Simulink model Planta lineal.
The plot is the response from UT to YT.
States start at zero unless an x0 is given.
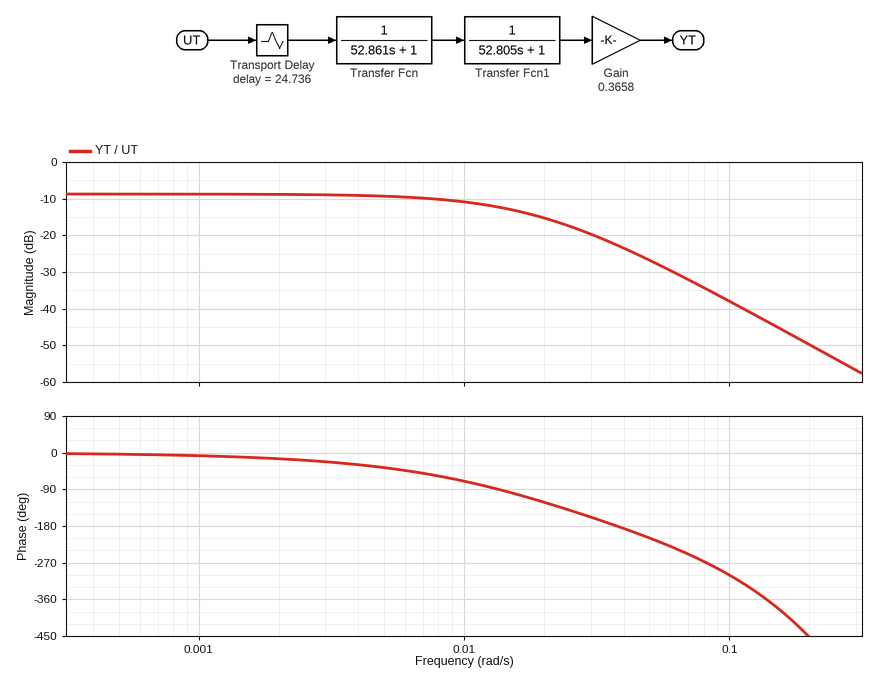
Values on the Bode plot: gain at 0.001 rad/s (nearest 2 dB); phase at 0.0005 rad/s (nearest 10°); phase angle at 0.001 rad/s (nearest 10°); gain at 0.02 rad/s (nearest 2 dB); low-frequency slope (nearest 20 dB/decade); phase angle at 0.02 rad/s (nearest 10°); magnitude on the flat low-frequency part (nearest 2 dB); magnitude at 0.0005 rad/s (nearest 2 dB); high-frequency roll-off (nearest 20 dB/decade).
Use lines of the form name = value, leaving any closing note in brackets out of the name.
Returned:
gain at 0.001 rad/s = -8 dB
phase at 0.0005 rad/s = 0°
phase angle at 0.001 rad/s = -10°
gain at 0.02 rad/s = -16 dB
low-frequency slope = 0 dB/decade
phase angle at 0.02 rad/s = -120°
magnitude on the flat low-frequency part = -8 dB
magnitude at 0.0005 rad/s = -8 dB
high-frequency roll-off = -40 dB/decade
